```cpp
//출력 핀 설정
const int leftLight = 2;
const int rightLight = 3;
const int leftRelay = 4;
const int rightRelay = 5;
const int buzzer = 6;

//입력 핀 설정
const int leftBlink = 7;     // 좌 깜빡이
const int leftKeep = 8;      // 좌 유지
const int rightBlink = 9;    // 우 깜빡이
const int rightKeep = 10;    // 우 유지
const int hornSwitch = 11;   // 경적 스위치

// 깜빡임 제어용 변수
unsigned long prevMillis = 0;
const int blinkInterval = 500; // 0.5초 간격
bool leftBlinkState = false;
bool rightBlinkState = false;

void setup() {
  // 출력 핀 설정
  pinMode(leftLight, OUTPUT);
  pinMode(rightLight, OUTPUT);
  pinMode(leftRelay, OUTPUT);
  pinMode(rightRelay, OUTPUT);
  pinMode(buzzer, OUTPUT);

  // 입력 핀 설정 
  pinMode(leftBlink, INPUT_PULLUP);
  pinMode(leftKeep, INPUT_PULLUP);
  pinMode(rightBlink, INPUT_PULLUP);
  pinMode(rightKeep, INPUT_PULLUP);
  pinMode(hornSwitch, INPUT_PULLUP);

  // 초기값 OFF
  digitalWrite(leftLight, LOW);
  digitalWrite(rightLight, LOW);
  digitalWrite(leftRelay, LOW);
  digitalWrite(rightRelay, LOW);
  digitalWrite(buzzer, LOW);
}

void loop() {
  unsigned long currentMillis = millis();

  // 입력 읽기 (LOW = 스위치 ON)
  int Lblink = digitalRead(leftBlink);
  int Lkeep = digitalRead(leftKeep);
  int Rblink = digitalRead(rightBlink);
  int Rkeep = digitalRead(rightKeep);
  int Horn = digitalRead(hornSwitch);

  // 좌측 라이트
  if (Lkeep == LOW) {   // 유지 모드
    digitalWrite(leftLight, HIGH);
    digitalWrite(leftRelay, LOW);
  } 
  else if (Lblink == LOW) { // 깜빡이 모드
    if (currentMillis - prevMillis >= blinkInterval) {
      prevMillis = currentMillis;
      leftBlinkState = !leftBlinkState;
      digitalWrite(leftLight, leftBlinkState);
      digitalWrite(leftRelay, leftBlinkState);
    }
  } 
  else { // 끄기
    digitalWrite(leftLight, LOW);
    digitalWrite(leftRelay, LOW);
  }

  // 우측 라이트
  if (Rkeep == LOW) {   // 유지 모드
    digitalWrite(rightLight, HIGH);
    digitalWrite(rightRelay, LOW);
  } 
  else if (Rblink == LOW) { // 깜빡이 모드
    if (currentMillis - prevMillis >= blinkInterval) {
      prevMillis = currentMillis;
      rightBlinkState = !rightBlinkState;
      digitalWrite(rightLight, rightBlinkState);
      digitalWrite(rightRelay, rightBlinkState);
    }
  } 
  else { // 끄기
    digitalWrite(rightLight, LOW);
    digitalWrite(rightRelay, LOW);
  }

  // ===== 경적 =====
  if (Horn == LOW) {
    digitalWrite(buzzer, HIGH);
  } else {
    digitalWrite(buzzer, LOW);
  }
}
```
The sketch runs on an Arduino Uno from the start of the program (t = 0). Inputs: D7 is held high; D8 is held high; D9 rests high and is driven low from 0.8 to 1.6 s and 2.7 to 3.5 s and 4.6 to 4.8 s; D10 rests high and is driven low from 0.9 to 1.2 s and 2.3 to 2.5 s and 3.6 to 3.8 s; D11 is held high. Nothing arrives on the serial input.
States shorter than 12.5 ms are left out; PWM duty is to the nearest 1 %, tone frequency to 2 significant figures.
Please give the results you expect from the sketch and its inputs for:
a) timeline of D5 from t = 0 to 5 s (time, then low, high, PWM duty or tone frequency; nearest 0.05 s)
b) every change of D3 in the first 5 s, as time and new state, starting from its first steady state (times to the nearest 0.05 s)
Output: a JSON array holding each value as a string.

["0 s low; 0.8 s high; 0.9 s low; 2.7 s high; 3.2 s low; 4.6 s high; 4.8 s low", "0 s low; 0.8 s high; 1.3 s low; 2.3 s high; 2.5 s low; 2.7 s high; 3.2 s low; 3.6 s high; 3.8 s low; 4.6 s high; 4.8 s low"]
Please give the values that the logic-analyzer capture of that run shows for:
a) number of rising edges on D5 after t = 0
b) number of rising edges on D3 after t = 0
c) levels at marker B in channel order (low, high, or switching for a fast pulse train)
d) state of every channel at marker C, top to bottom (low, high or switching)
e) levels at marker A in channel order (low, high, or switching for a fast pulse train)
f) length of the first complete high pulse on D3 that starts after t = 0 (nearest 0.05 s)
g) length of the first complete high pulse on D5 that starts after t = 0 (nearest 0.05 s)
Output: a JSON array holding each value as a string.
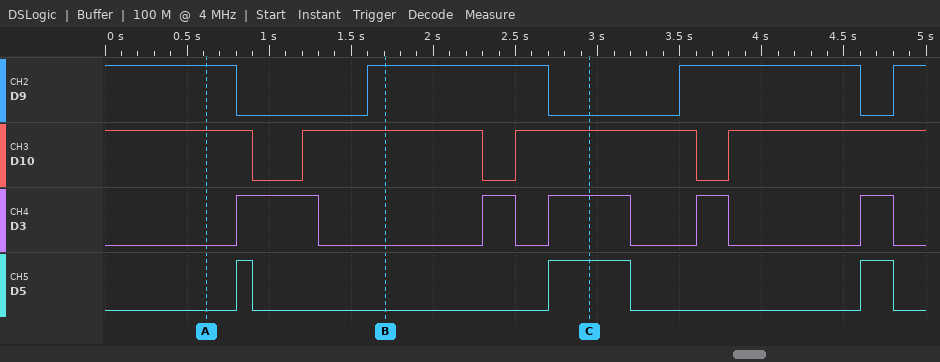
["3", "5", "D9 high, D10 high, D3 low, D5 low", "D9 low, D10 high, D3 high, D5 high", "D9 high, D10 high, D3 low, D5 low", "0.50 s", "0.10 s"]
